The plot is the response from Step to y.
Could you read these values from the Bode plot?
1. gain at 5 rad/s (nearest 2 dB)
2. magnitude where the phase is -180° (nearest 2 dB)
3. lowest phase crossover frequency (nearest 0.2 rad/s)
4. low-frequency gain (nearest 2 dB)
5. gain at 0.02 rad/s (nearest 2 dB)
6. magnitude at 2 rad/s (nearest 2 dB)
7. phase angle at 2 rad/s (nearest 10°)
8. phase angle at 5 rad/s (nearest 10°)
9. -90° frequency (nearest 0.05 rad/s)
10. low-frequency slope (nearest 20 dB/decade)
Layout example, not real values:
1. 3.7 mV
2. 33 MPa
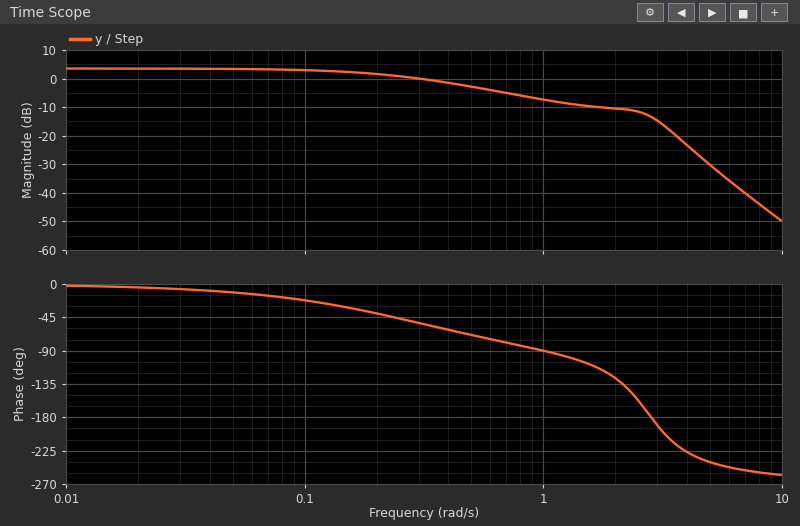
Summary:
1. -30 dB
2. -14 dB
3. 2.8 rad/s
4. 4 dB
5. 4 dB
6. -10 dB
7. -130°
8. -240°
9. 1.00 rad/s
10. 0 dB/decade
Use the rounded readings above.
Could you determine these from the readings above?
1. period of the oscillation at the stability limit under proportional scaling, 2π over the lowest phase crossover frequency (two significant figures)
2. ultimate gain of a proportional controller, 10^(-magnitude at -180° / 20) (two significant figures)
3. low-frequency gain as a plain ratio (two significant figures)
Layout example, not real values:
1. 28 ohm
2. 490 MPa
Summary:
1. 2.2 s
2. 5.0
3. 1.6
